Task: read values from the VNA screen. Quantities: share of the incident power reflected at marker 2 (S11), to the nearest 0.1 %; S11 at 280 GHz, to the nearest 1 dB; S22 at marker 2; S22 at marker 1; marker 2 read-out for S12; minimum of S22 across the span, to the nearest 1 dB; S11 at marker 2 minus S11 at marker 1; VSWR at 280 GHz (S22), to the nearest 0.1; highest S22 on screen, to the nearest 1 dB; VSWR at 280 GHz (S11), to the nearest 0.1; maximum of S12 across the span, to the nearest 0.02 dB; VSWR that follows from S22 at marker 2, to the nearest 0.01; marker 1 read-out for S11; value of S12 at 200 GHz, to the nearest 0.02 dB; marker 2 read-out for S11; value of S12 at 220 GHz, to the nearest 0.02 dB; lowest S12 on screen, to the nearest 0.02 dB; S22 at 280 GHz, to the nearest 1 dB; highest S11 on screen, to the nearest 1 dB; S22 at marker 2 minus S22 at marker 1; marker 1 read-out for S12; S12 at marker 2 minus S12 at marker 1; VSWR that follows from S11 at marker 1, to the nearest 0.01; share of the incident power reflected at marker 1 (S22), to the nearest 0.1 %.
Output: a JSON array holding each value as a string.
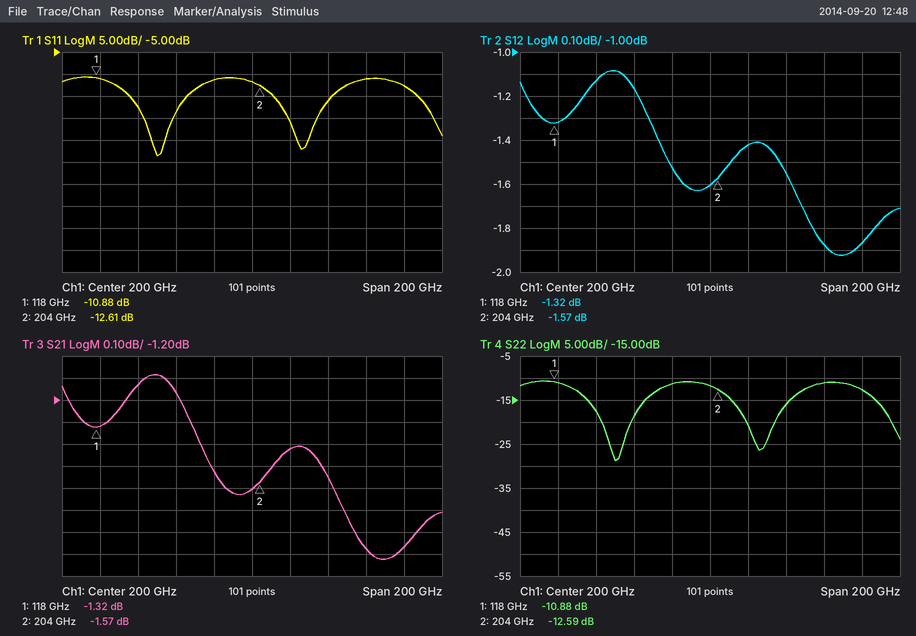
["5.5 %", "-13 dB", "-12.59 dB", "-10.88 dB", "-1.57 dB", "-29 dB", "-1.73 dB", "1.6", "-11 dB", "1.6", "-1.08 dB", "1.61", "-10.88 dB", "-1.60 dB", "-12.61 dB", "-1.42 dB", "-1.92 dB", "-13 dB", "-11 dB", "-1.71 dB", "-1.32 dB", "-0.25 dB", "1.80", "8.2 %"]
